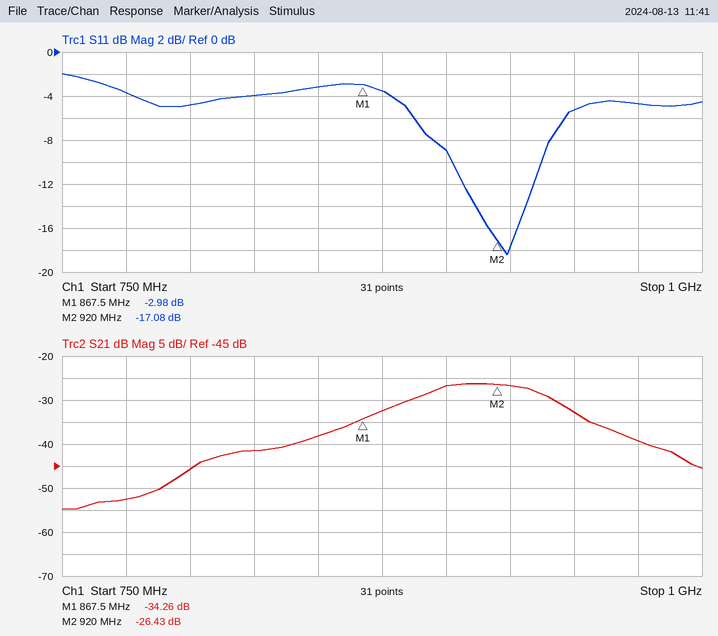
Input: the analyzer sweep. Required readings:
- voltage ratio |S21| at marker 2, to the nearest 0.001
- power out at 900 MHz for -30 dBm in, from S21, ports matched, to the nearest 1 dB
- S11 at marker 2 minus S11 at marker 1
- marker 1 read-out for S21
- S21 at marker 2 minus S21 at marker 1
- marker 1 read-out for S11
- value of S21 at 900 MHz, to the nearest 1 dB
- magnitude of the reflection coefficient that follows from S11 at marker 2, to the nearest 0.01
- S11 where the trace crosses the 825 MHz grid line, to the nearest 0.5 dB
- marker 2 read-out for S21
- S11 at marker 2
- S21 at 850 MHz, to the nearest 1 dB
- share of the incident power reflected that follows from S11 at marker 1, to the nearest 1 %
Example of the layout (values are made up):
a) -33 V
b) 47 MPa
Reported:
a) 0.048
b) -57 dBm
c) -14.10 dB
d) -34.26 dB
e) 7.83 dB
f) -2.98 dB
g) -27 dB
h) 0.14
i) -4.0 dB
j) -26.43 dB
k) -17.08 dB
l) -38 dB
m) 50 %
